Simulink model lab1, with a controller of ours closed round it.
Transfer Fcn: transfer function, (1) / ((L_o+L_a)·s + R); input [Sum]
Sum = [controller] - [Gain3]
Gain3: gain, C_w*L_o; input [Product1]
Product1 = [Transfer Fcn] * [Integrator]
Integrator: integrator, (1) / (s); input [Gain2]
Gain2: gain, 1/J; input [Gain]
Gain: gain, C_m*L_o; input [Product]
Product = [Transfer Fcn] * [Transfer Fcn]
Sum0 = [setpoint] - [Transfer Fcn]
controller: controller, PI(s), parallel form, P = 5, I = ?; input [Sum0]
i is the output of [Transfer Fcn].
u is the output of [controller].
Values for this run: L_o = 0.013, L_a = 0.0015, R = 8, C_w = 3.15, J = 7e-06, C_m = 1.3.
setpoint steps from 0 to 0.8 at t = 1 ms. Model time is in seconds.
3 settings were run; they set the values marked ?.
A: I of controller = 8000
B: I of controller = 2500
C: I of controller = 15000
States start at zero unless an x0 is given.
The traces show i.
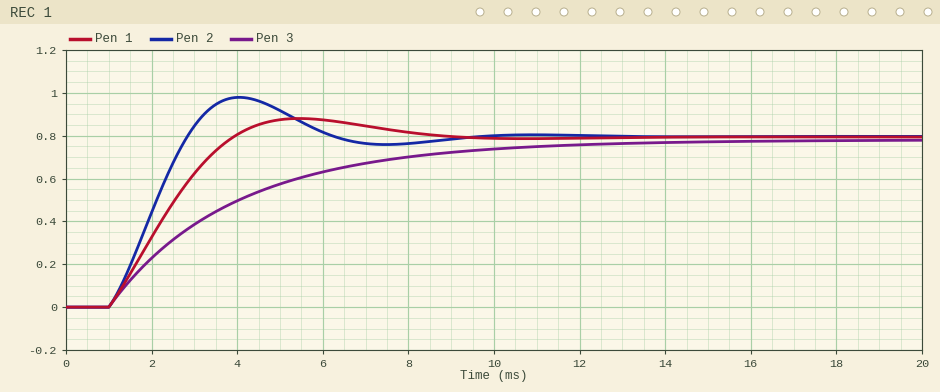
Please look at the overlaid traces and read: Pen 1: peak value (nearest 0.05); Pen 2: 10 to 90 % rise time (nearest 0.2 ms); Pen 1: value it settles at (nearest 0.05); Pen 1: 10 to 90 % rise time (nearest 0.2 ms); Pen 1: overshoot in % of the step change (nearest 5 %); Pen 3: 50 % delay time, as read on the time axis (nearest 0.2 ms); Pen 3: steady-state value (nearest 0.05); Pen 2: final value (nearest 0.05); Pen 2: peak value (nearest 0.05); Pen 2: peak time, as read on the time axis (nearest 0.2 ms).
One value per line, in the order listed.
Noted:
0.90
1.4 ms
0.80
2.2 ms
10 %
3.0 ms
0.80
0.80
1.00
4.0 ms
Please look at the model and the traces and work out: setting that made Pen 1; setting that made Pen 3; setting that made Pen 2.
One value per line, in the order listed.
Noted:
A
B
C
